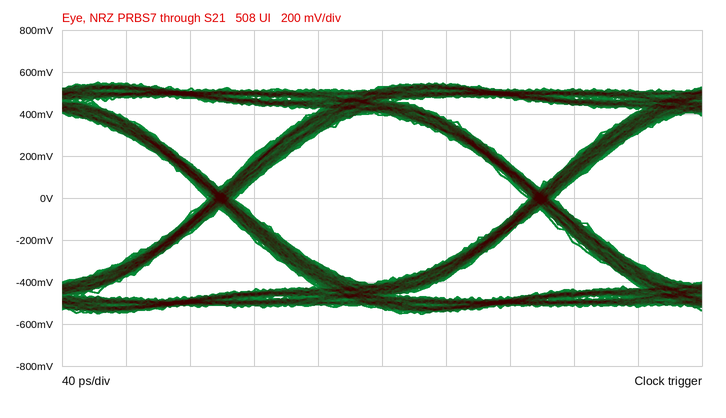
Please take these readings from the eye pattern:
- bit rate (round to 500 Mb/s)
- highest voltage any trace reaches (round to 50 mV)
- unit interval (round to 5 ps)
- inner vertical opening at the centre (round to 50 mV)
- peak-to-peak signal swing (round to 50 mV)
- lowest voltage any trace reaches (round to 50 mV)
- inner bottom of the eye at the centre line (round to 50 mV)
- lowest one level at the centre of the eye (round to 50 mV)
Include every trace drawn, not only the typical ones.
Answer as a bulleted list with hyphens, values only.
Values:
- 5.0 Gb/s
- 550 mV
- 200 ps
- 800 mV
- 1.10 V
- -550 mV
- -400 mV
- 400 mV
